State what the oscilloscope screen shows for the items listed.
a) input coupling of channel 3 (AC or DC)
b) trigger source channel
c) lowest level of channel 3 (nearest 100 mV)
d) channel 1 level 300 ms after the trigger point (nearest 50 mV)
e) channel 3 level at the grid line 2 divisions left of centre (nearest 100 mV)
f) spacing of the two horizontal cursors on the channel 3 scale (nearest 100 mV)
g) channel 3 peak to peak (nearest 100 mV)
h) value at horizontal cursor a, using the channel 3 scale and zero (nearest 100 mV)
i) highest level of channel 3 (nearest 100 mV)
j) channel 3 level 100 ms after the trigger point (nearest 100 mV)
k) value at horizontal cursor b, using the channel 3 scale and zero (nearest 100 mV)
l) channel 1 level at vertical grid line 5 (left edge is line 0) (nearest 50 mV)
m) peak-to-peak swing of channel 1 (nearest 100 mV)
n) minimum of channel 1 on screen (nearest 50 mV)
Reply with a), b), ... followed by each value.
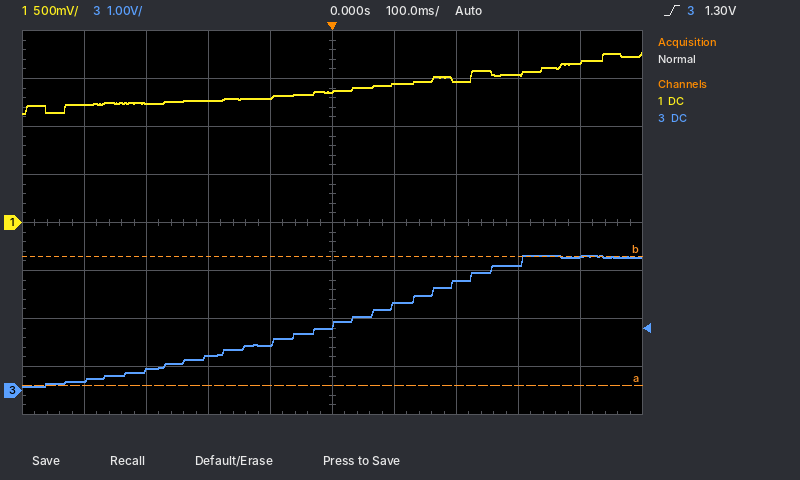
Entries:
a) DC
b) channel 3
c) 100 mV
d) 1.55 V
e) 700 mV
f) 2.7 V
g) 2.7 V
h) 100 mV
i) 2.8 V
j) 1.8 V
k) 2.8 V
l) 1.35 V
m) 600 mV
n) 1.15 V
